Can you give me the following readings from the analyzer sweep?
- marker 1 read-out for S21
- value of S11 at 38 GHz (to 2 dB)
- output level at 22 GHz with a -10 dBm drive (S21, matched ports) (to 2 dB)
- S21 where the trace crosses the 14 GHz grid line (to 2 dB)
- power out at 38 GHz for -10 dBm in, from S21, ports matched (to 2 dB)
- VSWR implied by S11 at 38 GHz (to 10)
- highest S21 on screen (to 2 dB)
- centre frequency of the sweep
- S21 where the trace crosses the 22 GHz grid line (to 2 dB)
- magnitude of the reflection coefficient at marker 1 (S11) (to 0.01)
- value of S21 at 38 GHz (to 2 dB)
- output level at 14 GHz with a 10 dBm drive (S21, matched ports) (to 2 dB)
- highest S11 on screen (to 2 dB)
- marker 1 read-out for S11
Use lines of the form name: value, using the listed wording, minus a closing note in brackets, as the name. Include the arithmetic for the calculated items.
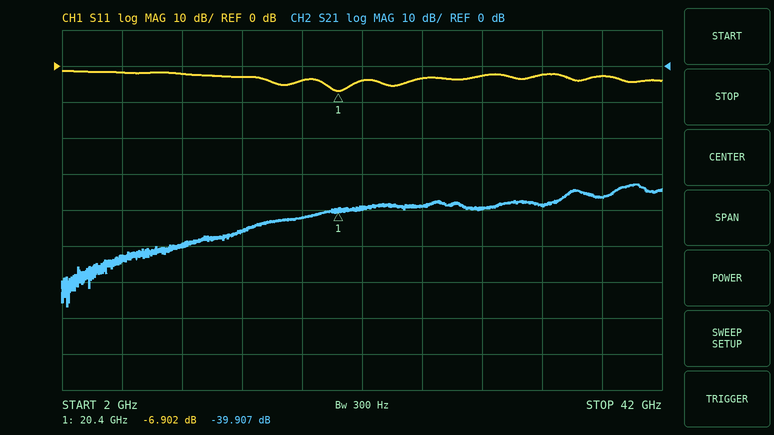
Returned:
marker 1 read-out for S21: -39.907 dB
value of S11 at 38 GHz: -2 dB
output level at 22 GHz with a -10 dBm drive (S21, matched ports): -10 dBm + (-40 dB) = -50 dBm
S21 where the trace crosses the 14 GHz grid line: -46 dB
power out at 38 GHz for -10 dBm in, from S21, ports matched: -10 dBm + (-36 dB) = -46 dBm
VSWR implied by S11 at 38 GHz: |Γ| = 10^(-2/20) = 0.7943; VSWR = (1 + 0.7943)/(1 − 0.7943) ≈ 8.72, so 10 to the nearest 10
highest S21 on screen: -32 dB
centre frequency of the sweep: 22 GHz
S21 where the trace crosses the 22 GHz grid line: -40 dB
magnitude of the reflection coefficient at marker 1 (S11): 10^(-6.902/20) ≈ 0.45
value of S21 at 38 GHz: -36 dB
output level at 14 GHz with a 10 dBm drive (S21, matched ports): 10 dBm + (-46 dB) = -36 dBm
highest S11 on screen: -2 dB
marker 1 read-out for S11: -6.902 dB
